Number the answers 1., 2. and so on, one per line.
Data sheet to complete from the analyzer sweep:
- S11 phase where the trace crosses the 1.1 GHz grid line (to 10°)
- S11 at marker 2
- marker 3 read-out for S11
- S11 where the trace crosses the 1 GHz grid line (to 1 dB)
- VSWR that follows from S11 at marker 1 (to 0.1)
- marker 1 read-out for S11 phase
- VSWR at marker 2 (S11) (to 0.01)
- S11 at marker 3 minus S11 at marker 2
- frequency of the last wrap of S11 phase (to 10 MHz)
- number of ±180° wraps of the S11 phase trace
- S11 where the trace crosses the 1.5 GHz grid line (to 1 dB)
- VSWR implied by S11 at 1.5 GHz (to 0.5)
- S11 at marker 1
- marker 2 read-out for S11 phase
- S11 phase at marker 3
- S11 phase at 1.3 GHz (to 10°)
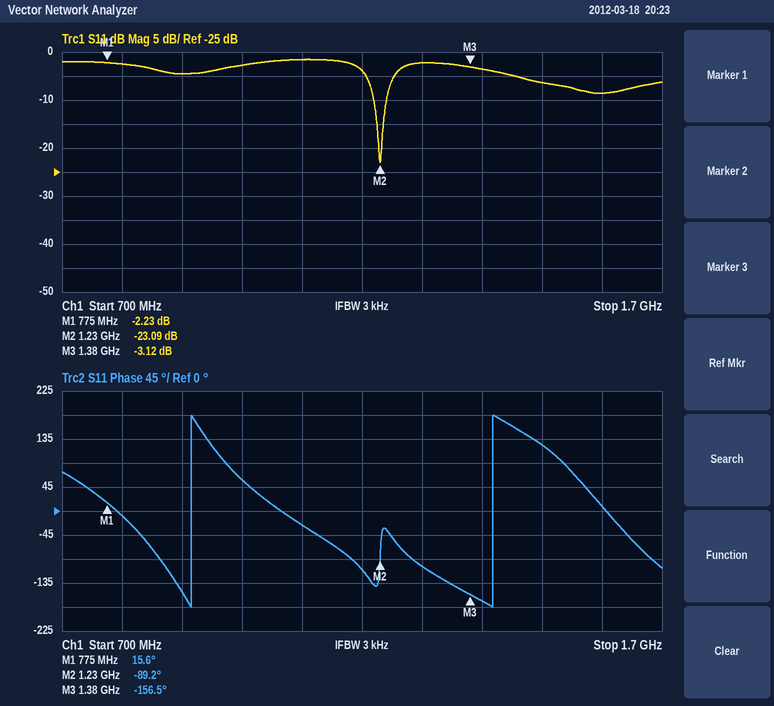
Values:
1. -30°
2. -23.09 dB
3. -3.12 dB
4. -3 dB
5. 7.8
6. 15.6°
7. 1.15
8. 19.97 dB
9. 1.42 GHz
10. 2
11. -6 dB
12. 3.0
13. -2.23 dB
14. -89.2°
15. -156.5°
16. -100°
